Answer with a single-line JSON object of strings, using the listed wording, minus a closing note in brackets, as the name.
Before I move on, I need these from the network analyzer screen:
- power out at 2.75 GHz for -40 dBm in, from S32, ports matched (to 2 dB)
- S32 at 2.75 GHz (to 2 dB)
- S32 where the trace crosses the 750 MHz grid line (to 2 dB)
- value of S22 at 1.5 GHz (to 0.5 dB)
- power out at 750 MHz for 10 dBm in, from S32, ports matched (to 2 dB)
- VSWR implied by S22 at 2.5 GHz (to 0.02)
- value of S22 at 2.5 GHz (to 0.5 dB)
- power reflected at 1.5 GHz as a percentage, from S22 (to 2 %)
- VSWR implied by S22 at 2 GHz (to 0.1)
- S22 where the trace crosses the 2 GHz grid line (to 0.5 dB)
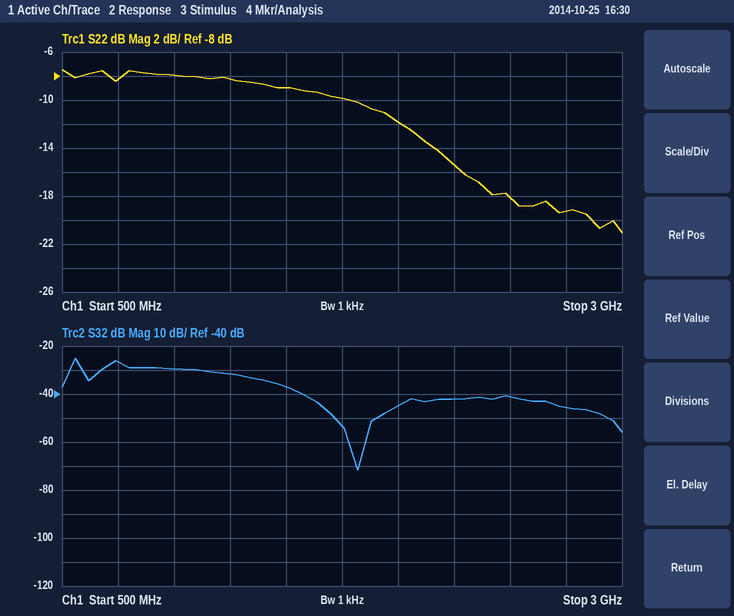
{"power out at 2.75 GHz for -40 dBm in, from S32, ports matched": "-86 dBm", "S32 at 2.75 GHz": "-46 dB", "S32 where the trace crosses the 750 MHz grid line": "-26 dB", "value of S22 at 1.5 GHz": "-9.0 dB", "power out at 750 MHz for 10 dBm in, from S32, ports matched": "-16 dBm", "VSWR implied by S22 at 2.5 GHz": "1.28", "value of S22 at 2.5 GHz": "-18.0 dB", "power reflected at 1.5 GHz as a percentage, from S22": "12 %", "VSWR implied by S22 at 2 GHz": "1.7", "S22 where the trace crosses the 2 GHz grid line": "-12.0 dB"}
